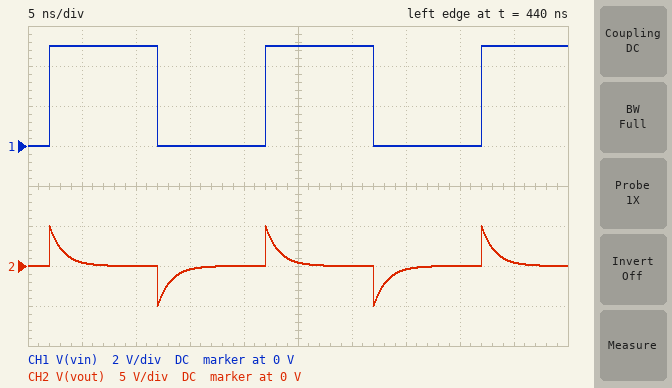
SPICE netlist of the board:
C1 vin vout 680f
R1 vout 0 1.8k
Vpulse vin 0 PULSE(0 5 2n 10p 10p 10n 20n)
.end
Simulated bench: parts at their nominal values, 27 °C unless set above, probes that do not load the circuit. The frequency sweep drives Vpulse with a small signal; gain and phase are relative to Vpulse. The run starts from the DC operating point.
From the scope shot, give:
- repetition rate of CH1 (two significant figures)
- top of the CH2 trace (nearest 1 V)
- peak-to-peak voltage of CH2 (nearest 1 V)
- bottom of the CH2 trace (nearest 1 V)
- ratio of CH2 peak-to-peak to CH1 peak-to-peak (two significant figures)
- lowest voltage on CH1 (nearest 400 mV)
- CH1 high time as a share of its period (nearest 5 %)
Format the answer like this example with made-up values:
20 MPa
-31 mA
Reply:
50 MHz
5 V
10 V
-5 V
2.0
0 V
50 %
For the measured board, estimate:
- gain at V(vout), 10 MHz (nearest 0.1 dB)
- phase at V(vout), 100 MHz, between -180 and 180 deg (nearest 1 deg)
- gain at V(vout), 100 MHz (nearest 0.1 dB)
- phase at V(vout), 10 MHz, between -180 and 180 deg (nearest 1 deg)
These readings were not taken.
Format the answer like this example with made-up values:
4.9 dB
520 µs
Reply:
-22.3 dB
52 deg
-4.3 dB
86 deg
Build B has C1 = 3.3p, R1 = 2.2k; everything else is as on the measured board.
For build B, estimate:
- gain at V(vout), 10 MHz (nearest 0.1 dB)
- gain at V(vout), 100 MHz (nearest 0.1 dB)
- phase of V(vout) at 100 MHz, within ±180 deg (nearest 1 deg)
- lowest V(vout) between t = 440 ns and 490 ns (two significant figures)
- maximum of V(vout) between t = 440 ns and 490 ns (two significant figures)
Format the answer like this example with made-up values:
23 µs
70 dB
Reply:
-7.6 dB
-0.2 dB
12 deg
-4.0 V
4.0 V
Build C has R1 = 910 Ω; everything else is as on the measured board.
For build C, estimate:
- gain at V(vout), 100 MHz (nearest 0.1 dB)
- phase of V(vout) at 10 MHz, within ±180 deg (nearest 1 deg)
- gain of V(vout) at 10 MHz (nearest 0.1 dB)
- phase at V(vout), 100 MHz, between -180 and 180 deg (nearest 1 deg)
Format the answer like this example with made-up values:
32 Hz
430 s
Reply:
-8.8 dB
88 deg
-28.2 dB
69 deg
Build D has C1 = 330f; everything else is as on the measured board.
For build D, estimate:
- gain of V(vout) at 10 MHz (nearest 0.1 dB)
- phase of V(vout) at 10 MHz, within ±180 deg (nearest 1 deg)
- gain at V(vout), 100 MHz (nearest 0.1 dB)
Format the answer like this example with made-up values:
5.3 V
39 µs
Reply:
-28.6 dB
88 deg
-9.1 dB
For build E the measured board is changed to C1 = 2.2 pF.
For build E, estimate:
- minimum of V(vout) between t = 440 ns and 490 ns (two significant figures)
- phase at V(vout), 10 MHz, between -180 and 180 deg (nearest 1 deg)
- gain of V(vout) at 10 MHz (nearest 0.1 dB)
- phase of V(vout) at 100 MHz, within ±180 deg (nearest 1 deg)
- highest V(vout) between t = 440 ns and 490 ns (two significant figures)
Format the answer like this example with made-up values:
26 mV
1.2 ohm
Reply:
-4.6 V
76 deg
-12.3 dB
22 deg
4.6 V
